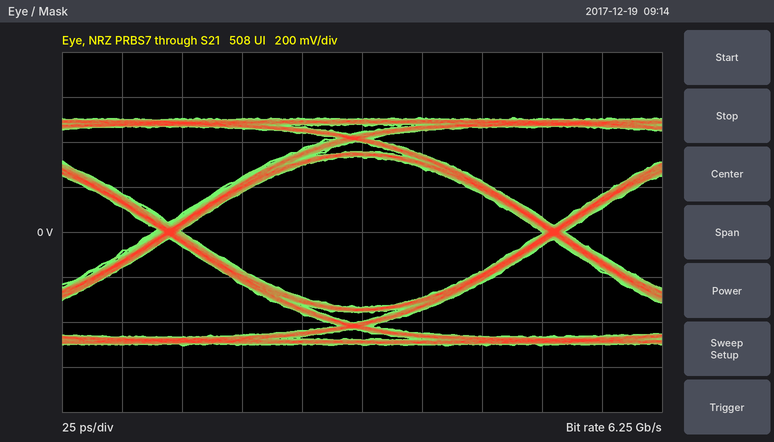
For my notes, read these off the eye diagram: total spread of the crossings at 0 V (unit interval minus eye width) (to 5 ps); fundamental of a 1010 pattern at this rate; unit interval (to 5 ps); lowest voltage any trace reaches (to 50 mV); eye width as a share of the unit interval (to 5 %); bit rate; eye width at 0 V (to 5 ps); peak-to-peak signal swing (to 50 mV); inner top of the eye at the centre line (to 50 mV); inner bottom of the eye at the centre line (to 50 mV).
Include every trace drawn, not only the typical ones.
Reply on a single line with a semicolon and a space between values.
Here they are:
10 ps; 3.125 GHz; 160 ps; -500 mV; 95 %; 6.25 Gb/s; 150 ps; 1.00 V; 350 mV; -350 mV
